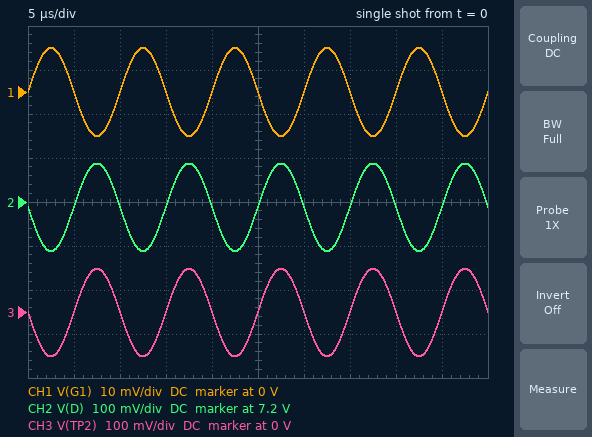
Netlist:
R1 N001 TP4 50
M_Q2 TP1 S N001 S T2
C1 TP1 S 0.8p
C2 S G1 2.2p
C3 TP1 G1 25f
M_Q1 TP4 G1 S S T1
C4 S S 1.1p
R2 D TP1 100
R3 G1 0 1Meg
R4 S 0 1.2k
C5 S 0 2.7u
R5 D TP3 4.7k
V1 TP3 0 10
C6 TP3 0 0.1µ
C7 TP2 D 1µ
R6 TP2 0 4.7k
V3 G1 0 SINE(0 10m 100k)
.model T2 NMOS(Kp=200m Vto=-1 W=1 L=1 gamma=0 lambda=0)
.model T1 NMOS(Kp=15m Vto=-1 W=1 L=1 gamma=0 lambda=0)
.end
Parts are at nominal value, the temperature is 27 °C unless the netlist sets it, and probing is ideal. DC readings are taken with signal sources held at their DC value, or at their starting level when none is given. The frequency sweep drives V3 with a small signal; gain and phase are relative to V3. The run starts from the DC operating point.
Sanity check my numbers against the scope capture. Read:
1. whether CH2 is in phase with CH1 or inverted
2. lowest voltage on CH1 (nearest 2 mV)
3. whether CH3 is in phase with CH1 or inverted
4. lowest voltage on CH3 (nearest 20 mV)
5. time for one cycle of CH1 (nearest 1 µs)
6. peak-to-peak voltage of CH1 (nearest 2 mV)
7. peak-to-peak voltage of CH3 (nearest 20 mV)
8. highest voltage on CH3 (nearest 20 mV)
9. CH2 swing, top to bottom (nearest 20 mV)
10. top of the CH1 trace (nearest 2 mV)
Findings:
inverted
-10 mV
inverted
-100 mV
10 µs
20 mV
200 mV
100 mV
200 mV
10 mV
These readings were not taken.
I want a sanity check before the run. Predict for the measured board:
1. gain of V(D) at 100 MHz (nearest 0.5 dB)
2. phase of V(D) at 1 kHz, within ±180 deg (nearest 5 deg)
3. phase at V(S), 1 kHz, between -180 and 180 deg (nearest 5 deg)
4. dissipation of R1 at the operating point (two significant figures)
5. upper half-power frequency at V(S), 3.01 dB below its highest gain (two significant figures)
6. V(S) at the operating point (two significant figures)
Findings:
16.0 dB
-165 deg
-75 deg
18 µW
300 Hz
720 mV
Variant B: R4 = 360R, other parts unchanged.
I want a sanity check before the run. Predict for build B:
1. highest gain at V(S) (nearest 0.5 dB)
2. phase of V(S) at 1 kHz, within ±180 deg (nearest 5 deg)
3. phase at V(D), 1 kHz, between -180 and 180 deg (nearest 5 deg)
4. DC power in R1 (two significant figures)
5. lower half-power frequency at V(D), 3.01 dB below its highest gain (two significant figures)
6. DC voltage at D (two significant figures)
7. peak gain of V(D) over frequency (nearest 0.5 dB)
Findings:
-3.0 dB
-60 deg
-160 deg
120 µW
510 Hz
2.8 V
24.0 dB
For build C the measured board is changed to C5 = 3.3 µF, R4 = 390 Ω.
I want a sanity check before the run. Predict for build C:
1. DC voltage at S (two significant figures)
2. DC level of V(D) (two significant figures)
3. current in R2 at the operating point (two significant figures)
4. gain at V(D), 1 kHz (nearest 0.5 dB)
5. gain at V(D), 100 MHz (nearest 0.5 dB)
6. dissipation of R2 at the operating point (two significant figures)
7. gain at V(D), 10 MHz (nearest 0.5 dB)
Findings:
560 mV
3.2 V
1.4 mA
23.0 dB
19.5 dB
210 µW
23.5 dB
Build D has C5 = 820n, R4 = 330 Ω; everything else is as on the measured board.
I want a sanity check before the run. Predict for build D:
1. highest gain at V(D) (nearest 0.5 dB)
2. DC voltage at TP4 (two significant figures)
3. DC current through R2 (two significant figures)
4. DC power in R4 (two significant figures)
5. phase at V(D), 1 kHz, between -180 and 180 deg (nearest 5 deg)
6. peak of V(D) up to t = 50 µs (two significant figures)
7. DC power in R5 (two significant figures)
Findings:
24.5 dB
1.3 V
1.6 mA
870 µW
-150 deg
2.5 V
12 mW
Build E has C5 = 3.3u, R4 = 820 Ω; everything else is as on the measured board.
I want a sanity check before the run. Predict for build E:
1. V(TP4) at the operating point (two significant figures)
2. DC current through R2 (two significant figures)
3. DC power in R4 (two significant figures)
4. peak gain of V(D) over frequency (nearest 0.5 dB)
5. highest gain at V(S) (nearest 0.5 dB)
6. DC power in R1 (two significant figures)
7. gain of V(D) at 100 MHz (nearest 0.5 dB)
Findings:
1.5 V
820 µA
550 µW
21.5 dB
-2.0 dB
33 µW
17.0 dB
